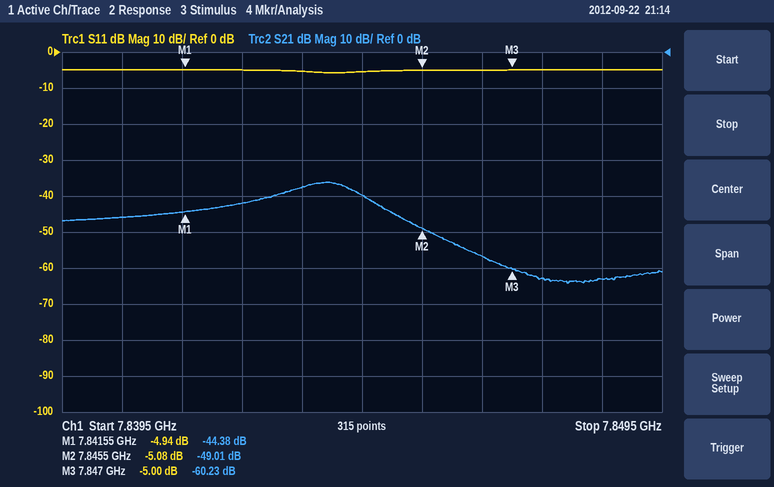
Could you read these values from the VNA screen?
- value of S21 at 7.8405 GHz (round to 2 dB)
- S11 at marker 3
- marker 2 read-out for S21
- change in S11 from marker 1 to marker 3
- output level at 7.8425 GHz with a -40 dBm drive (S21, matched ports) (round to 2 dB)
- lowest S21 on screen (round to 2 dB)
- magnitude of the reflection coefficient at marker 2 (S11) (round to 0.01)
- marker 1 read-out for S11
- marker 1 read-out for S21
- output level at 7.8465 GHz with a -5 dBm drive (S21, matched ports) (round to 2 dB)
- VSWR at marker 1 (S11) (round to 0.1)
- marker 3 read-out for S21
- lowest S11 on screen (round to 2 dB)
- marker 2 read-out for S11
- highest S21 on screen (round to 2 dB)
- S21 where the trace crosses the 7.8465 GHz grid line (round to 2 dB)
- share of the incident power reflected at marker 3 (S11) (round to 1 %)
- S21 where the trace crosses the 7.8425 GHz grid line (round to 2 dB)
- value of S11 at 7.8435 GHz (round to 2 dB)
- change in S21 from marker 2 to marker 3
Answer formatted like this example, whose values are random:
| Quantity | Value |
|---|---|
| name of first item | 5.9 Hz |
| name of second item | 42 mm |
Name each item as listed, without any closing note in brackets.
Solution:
| Quantity | Value |
|---|---|
| value of S21 at 7.8405 GHz | -46 dB |
| S11 at marker 3 | -5.00 dB |
| marker 2 read-out for S21 | -49.01 dB |
| change in S11 from marker 1 to marker 3 | -0.06 dB |
| output level at 7.8425 GHz with a -40 dBm drive (S21, matched ports) | -82 dBm |
| lowest S21 on screen | -64 dB |
| magnitude of the reflection coefficient at marker 2 (S11) | 0.56 |
| marker 1 read-out for S11 | -4.94 dB |
| marker 1 read-out for S21 | -44.38 dB |
| output level at 7.8465 GHz with a -5 dBm drive (S21, matched ports) | -62 dBm |
| VSWR at marker 1 (S11) | 3.6 |
| marker 3 read-out for S21 | -60.23 dB |
| lowest S11 on screen | -6 dB |
| marker 2 read-out for S11 | -5.08 dB |
| highest S21 on screen | -36 dB |
| S21 where the trace crosses the 7.8465 GHz grid line | -56 dB |
| share of the incident power reflected at marker 3 (S11) | 32 % |
| S21 where the trace crosses the 7.8425 GHz grid line | -42 dB |
| value of S11 at 7.8435 GHz | -6 dB |
| change in S21 from marker 2 to marker 3 | -11.22 dB |
